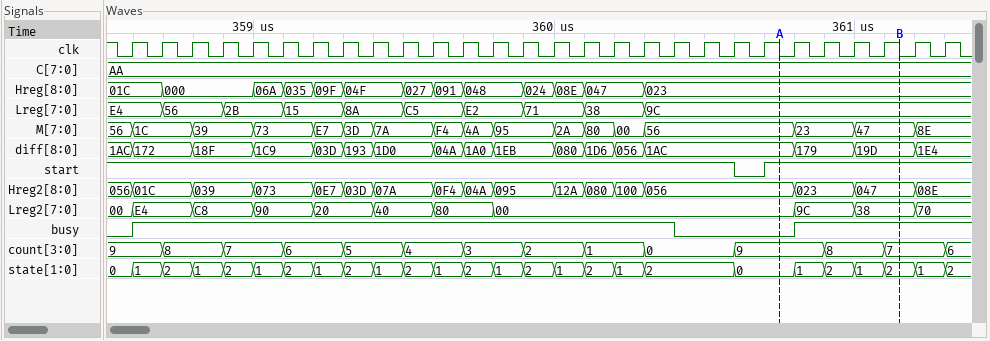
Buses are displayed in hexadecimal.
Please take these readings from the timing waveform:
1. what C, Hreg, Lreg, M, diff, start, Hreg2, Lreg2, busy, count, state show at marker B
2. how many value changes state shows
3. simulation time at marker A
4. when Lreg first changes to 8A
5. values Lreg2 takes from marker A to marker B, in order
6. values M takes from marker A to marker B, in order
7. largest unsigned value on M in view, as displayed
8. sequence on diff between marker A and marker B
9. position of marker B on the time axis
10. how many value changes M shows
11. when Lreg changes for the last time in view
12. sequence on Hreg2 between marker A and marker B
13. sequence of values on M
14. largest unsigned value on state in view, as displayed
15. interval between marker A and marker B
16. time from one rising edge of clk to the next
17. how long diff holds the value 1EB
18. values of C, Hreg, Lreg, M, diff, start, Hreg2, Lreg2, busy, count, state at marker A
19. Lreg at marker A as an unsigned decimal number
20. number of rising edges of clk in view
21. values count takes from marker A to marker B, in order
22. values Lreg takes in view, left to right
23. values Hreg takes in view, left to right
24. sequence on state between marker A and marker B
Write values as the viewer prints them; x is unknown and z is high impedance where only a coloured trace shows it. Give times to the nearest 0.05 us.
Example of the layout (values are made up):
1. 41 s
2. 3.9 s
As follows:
1. C=AA, Hreg=023, Lreg=9C, M=47, diff=19D, start=1, Hreg2=047, Lreg2=38, busy=1, count=7, state=2
2. 25
3. 360.75 us
4. 359.3 us
5. 00, 9C, 38
6. 56, 23, 47
7. F4
8. 1AC, 179, 19D
9. 361.15 us
10. 16
11. 360.3 us
12. 056, 023, 047
13. 56, 1C, 39, 73, E7, 3D, 7A, F4, 4A, 95, 2A, 80, 00, 56, 23, 47, 8E
14. 2
15. 0.4 us
16. 0.1 us
17. 0.2 us
18. C=AA, Hreg=023, Lreg=9C, M=56, diff=1AC, start=1, Hreg2=056, Lreg2=00, busy=0, count=9, state=0
19. 156
20. 28
21. 9, 8, 7
22. E4, 56, 2B, 15, 8A, C5, E2, 71, 38, 9C
23. 01C, 000, 06A, 035, 09F, 04F, 027, 091, 048, 024, 08E, 047, 023
24. 0, 1, 2, 1, 2
